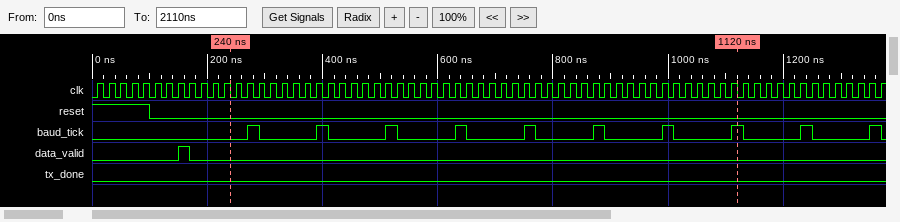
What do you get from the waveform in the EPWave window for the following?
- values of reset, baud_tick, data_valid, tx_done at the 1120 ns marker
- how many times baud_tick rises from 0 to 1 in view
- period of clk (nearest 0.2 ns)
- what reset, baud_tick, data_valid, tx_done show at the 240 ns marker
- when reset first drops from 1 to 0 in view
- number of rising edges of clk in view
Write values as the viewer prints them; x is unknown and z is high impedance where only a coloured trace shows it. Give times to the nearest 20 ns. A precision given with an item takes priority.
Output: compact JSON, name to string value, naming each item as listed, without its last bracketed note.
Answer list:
{"values of reset, baud_tick, data_valid, tx_done at the 1120 ns marker": "reset=0, baud_tick=1, data_valid=0, tx_done=0", "how many times baud_tick rises from 0 to 1 in view": "10", "period of clk": "20 ns", "what reset, baud_tick, data_valid, tx_done show at the 240 ns marker": "reset=0, baud_tick=0, data_valid=0, tx_done=0", "when reset first drops from 1 to 0 in view": "100 ns", "number of rising edges of clk in view": "69"}
